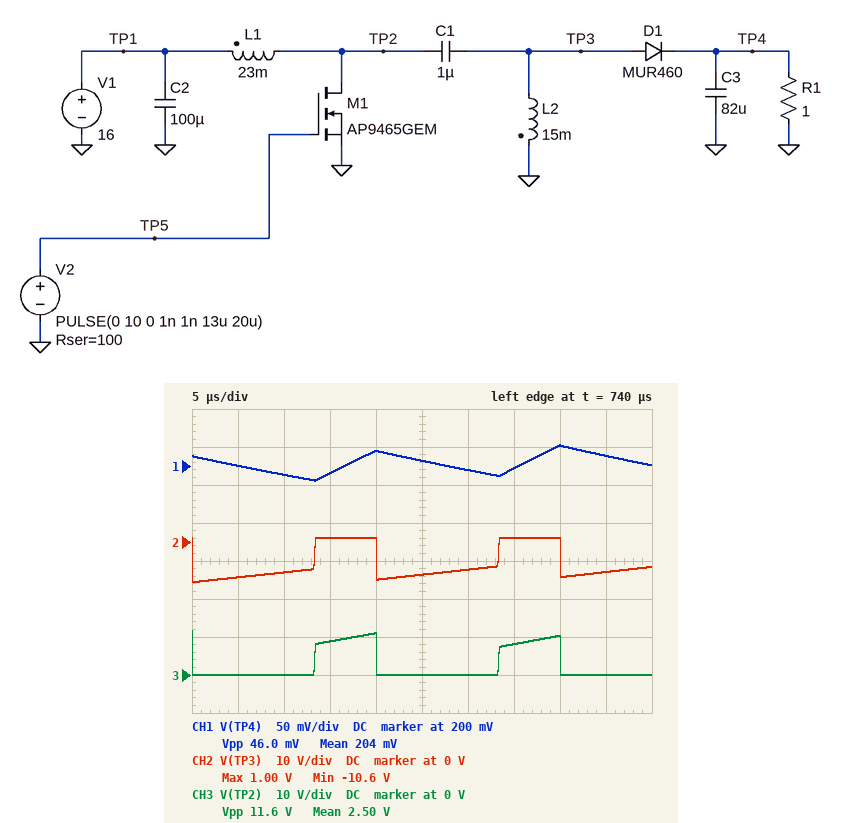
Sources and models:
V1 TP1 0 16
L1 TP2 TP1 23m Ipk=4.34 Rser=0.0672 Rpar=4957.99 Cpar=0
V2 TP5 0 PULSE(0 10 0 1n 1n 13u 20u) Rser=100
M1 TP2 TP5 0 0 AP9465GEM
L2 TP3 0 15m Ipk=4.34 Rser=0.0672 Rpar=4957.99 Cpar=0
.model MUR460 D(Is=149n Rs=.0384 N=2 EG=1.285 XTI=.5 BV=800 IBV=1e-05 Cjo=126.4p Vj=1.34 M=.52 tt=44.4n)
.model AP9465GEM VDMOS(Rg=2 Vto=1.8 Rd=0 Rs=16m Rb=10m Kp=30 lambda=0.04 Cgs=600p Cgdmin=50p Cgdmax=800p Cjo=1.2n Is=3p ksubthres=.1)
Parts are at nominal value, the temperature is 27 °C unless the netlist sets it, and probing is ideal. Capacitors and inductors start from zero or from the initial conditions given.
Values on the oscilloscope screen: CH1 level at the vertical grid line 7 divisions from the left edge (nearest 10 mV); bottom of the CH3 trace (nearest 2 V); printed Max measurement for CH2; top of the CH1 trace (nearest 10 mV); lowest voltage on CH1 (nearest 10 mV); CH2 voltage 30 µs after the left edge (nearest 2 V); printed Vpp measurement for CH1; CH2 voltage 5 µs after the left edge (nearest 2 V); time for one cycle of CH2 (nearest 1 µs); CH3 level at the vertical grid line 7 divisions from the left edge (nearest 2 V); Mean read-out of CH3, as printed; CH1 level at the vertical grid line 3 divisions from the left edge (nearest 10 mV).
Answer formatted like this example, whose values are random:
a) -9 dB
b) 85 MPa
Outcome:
a) 200 mV
b) 0 V
c) 1.00 V
d) 230 mV
e) 180 mV
f) -8 V
g) 46.0 mV
h) -10 V
i) 20 µs
j) 8 V
k) 2.50 V
l) 190 mV
